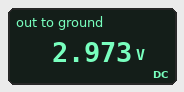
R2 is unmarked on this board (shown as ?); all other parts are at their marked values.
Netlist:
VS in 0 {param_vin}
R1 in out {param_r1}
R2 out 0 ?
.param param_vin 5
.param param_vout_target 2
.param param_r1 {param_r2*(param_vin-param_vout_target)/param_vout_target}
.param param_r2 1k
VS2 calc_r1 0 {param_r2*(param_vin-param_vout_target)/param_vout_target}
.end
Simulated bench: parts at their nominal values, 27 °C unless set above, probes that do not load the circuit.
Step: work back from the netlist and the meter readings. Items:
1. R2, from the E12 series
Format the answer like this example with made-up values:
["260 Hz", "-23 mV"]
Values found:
["2.2 kΩ"]
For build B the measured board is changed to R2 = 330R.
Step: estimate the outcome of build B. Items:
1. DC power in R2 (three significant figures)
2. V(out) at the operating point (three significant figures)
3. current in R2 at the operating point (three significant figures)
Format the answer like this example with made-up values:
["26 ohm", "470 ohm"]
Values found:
["2.46 mW", "902 mV", "2.73 mA"]
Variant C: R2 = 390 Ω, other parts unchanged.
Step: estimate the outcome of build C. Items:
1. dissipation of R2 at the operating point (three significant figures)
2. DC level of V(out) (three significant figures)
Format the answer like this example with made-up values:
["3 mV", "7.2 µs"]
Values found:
["2.73 mW", "1.03 V"]
